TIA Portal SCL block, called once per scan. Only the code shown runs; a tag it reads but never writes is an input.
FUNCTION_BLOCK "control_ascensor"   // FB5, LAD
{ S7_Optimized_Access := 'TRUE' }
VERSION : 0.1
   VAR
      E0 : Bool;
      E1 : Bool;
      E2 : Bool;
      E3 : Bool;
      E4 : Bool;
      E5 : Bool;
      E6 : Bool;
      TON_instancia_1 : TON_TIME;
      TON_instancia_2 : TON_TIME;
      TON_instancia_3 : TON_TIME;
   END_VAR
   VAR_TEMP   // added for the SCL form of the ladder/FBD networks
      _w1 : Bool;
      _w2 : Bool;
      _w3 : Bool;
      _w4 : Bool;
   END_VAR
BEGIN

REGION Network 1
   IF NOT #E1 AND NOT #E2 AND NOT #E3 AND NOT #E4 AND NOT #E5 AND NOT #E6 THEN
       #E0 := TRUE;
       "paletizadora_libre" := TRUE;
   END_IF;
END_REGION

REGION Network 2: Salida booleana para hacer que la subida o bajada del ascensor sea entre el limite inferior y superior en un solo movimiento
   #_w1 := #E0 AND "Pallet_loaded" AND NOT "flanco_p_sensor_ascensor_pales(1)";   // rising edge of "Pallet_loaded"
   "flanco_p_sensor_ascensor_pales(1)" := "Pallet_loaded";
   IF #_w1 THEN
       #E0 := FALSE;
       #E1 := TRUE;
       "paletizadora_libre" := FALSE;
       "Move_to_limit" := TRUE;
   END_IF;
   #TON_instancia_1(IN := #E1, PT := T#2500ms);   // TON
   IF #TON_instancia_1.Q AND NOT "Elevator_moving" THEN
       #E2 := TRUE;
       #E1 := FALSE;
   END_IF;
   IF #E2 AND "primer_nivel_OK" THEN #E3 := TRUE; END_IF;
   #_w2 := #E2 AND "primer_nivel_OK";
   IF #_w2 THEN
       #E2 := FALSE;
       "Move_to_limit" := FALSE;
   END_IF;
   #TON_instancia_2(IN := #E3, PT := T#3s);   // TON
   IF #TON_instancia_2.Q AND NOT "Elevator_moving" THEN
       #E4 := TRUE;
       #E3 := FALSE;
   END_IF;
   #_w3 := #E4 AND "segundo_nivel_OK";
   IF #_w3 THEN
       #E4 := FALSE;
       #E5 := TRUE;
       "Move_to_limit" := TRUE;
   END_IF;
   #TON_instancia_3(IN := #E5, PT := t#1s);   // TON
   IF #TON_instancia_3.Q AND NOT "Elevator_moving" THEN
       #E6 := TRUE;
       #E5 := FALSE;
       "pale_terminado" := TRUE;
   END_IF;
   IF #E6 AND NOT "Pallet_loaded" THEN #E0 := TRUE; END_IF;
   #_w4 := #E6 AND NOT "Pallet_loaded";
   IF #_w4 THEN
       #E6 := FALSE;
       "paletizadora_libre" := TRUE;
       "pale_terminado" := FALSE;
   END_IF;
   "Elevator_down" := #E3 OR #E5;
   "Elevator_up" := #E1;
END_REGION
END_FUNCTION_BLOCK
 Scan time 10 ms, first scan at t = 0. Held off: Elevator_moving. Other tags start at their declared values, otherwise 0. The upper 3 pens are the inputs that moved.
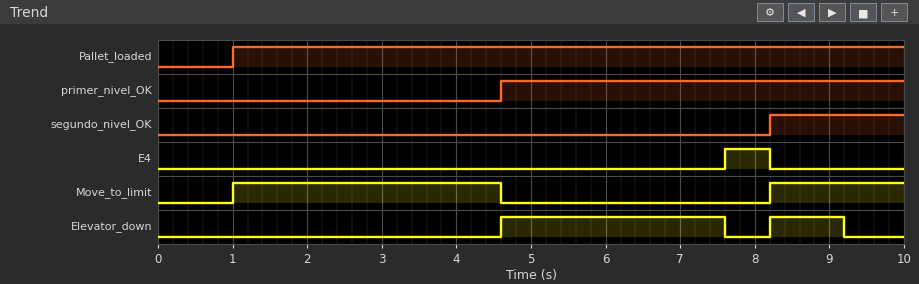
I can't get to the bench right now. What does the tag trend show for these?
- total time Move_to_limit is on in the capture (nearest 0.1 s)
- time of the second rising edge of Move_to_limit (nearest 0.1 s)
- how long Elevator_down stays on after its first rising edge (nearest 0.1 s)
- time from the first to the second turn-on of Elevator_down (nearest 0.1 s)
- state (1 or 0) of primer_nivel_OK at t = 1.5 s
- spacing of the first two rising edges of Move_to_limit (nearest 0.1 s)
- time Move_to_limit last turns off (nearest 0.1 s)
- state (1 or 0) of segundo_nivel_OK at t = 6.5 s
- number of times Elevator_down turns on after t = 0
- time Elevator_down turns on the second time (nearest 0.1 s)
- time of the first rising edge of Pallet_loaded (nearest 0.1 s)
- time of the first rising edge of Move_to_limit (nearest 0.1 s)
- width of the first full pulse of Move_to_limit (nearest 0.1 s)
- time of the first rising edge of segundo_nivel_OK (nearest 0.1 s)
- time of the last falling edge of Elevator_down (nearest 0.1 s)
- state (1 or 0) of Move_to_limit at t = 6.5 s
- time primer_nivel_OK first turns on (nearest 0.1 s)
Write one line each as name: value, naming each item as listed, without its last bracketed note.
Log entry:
total time Move_to_limit is on in the capture: 5.4 s
time of the second rising edge of Move_to_limit: 8.2 s
how long Elevator_down stays on after its first rising edge: 3.0 s
time from the first to the second turn-on of Elevator_down: 3.6 s
state (1 or 0) of primer_nivel_OK at t = 1.5 s: 0
spacing of the first two rising edges of Move_to_limit: 7.2 s
time Move_to_limit last turns off: 4.6 s
state (1 or 0) of segundo_nivel_OK at t = 6.5 s: 0
number of times Elevator_down turns on after t = 0: 2
time Elevator_down turns on the second time: 8.2 s
time of the first rising edge of Pallet_loaded: 1.0 s
time of the first rising edge of Move_to_limit: 1.0 s
width of the first full pulse of Move_to_limit: 3.6 s
time of the first rising edge of segundo_nivel_OK: 8.2 s
time of the last falling edge of Elevator_down: 9.2 s
state (1 or 0) of Move_to_limit at t = 6.5 s: 0
time primer_nivel_OK first turns on: 4.6 s
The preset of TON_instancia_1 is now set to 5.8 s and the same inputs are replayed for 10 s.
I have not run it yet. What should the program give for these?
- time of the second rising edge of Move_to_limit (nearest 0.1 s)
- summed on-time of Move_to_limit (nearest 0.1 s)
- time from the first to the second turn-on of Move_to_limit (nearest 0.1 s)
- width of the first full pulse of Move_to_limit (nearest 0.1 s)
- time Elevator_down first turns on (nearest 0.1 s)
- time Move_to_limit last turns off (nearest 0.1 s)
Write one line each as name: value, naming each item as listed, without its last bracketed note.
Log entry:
time of the second rising edge of Move_to_limit: 9.8 s
summed on-time of Move_to_limit: 6.0 s
time from the first to the second turn-on of Move_to_limit: 8.8 s
width of the first full pulse of Move_to_limit: 5.8 s
time Elevator_down first turns on: 6.8 s
time Move_to_limit last turns off: 6.8 s
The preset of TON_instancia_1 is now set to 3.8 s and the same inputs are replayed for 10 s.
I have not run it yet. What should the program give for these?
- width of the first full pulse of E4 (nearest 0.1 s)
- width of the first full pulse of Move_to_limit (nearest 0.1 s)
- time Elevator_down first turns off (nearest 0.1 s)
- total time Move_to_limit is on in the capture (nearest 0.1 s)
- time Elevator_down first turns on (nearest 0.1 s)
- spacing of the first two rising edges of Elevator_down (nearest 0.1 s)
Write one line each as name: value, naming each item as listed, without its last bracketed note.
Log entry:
width of the first full pulse of E4: 0.4 s
width of the first full pulse of Move_to_limit: 3.8 s
time Elevator_down first turns off: 7.8 s
total time Move_to_limit is on in the capture: 5.6 s
time Elevator_down first turns on: 4.8 s
spacing of the first two rising edges of Elevator_down: 3.4 s
